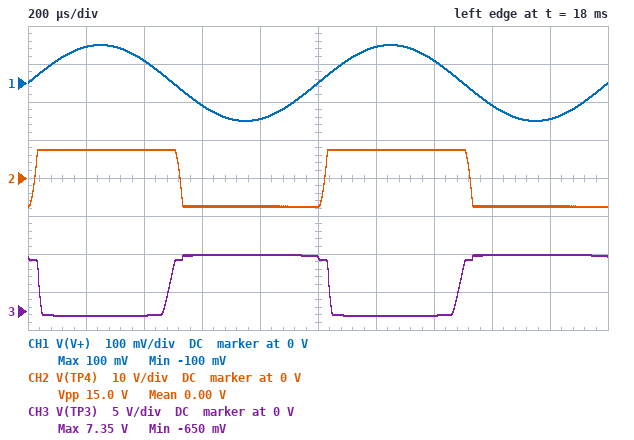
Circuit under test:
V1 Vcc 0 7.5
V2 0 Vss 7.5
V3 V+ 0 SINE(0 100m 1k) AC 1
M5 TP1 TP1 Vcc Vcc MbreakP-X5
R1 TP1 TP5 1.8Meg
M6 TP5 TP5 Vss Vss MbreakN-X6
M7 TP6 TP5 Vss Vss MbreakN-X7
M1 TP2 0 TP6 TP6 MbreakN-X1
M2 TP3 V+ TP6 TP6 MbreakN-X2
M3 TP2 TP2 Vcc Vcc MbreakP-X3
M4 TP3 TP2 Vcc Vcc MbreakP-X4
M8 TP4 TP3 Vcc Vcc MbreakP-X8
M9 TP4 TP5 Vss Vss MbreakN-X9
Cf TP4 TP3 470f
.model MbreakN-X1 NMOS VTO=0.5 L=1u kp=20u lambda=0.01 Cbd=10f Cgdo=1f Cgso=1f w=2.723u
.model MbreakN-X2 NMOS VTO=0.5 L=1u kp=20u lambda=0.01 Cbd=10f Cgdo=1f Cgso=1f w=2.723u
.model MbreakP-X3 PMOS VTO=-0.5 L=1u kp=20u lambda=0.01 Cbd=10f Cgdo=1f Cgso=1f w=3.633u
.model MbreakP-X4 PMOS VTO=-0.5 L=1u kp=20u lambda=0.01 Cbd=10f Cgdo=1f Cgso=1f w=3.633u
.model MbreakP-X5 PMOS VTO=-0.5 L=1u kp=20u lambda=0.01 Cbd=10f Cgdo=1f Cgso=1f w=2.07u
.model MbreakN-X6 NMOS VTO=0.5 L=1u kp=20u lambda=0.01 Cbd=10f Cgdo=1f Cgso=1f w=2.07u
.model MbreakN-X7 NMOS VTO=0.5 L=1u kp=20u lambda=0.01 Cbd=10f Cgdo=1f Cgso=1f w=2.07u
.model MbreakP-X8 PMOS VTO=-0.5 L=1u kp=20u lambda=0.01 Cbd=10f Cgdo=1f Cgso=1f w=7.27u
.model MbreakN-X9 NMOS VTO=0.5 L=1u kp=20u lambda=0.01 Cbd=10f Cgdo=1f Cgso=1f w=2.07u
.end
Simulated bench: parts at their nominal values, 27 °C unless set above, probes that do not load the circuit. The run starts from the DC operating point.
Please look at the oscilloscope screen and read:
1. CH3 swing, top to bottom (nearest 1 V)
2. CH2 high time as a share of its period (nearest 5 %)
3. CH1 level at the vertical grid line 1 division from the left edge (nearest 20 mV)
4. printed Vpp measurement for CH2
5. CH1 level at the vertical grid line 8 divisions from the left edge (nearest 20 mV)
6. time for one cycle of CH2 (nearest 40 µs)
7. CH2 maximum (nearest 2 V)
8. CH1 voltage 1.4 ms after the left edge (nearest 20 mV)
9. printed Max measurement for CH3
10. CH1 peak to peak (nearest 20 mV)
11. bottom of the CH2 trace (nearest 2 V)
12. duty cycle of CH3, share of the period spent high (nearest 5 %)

8 V
50 %
100 mV
15.0 V
-60 mV
1.00 ms
8 V
60 mV
7.35 V
200 mV
-8 V
55 %
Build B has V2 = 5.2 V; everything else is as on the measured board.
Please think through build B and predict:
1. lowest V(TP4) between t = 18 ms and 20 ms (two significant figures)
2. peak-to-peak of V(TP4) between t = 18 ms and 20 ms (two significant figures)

-5.2 V
13 V
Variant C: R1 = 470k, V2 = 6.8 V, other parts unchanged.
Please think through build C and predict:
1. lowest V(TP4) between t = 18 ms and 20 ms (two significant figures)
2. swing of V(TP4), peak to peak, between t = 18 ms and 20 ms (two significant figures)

-6.8 V
14 V
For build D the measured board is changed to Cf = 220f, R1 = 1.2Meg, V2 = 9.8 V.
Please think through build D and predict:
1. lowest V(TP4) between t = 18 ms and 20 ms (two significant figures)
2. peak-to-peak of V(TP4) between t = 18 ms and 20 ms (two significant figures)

-9.8 V
17 V
